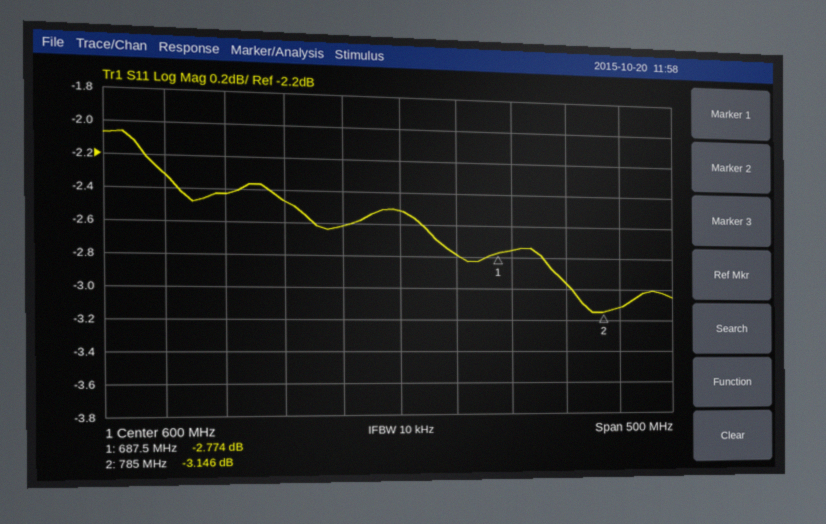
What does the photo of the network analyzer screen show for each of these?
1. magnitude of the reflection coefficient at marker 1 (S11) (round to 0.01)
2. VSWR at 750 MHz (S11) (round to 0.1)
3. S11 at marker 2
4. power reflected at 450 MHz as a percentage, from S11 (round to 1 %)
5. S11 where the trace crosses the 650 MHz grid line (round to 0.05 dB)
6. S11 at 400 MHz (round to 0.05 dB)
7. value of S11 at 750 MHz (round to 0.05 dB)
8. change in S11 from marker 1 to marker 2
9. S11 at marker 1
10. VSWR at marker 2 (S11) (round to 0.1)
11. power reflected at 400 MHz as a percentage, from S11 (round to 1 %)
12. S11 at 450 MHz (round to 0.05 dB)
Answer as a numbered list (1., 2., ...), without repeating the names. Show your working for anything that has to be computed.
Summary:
1. 10^(-2.774/20) ≈ 0.73
2. |Γ| = 10^(-2.95/20) = 0.7120; VSWR = (1 + 0.7120)/(1 − 0.7120) ≈ 5.9
3. -3.146 dB
4. 10^(-2.45/10) ≈ 57 %
5. -2.80 dB
6. -2.30 dB
7. -2.95 dB
8. -3.146 − (-2.774) = -0.372 dB
9. -2.774 dB
10. (1 + 0.6961)/(1 − 0.6961) ≈ 5.6
11. 10^(-2.3/10) ≈ 59 %
12. -2.45 dB
